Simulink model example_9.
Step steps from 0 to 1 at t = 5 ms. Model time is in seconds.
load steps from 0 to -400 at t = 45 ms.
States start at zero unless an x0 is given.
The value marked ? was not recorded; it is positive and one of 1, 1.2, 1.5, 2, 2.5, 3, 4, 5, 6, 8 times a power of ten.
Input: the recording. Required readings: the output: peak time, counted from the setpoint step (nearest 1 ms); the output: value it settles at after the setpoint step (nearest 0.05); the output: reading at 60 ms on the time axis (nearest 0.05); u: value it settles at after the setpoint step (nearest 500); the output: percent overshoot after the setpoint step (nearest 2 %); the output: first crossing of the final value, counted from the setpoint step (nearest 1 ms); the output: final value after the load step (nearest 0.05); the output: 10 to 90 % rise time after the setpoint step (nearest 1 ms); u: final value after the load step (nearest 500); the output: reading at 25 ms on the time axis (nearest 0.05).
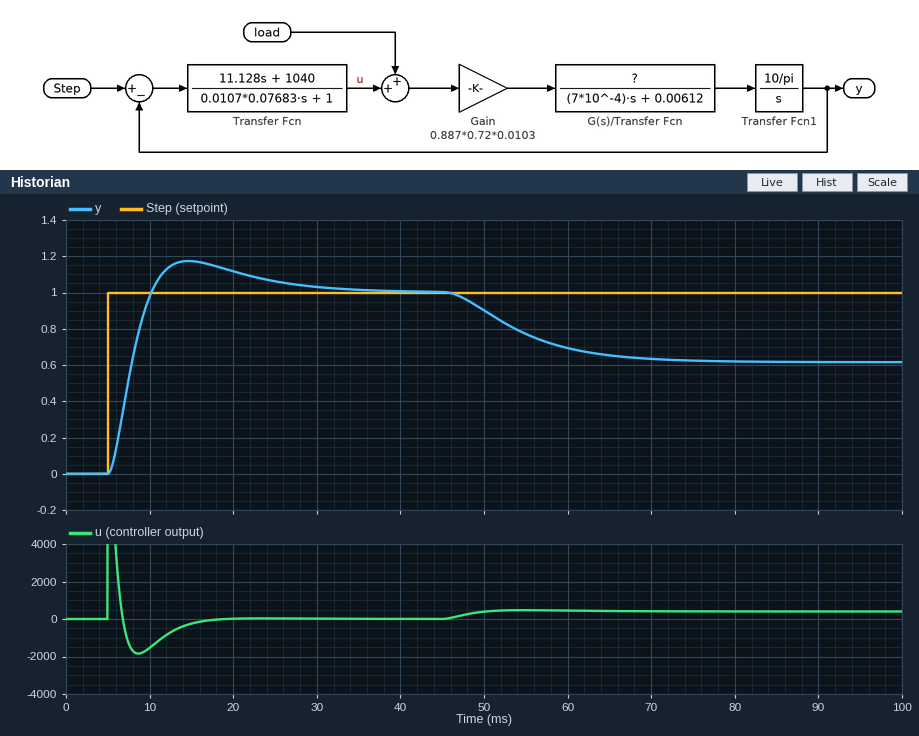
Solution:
10 ms
1.00
0.70
0
18 %
5 ms
0.60
4 ms
500
1.05
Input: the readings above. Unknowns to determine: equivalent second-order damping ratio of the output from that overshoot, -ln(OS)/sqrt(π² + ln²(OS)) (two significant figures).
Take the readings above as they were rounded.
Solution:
0.48
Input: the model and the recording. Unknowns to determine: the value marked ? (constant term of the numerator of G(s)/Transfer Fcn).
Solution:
1
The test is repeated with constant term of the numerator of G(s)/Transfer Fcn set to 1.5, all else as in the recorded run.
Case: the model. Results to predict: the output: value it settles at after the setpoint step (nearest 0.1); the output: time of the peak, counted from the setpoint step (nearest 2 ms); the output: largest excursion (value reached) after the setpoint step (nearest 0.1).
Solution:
1.0
6 ms
1.2
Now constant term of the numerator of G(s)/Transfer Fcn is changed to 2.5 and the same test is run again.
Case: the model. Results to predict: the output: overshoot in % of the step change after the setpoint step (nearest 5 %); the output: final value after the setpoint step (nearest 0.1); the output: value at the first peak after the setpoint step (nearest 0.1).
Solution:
20 %
1.0
1.2
